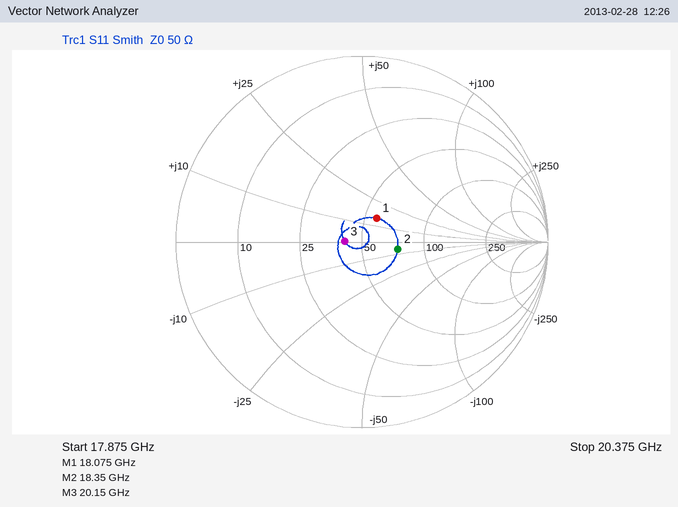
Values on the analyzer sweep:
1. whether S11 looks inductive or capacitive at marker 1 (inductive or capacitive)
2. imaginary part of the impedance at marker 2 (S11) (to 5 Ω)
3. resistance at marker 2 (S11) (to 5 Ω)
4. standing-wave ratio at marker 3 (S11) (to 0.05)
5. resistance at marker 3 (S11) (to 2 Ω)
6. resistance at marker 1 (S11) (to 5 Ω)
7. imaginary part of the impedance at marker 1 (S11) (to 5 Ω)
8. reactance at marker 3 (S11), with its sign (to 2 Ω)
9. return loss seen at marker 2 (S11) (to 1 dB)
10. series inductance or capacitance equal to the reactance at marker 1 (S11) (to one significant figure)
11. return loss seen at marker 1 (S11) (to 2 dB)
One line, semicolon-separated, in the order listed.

inductive; -5 Ω; 75 Ω; 1.20; 42 Ω; 55 Ω; +15 Ω; 0 Ω; 14 dB; 100 pH; 16 dB
